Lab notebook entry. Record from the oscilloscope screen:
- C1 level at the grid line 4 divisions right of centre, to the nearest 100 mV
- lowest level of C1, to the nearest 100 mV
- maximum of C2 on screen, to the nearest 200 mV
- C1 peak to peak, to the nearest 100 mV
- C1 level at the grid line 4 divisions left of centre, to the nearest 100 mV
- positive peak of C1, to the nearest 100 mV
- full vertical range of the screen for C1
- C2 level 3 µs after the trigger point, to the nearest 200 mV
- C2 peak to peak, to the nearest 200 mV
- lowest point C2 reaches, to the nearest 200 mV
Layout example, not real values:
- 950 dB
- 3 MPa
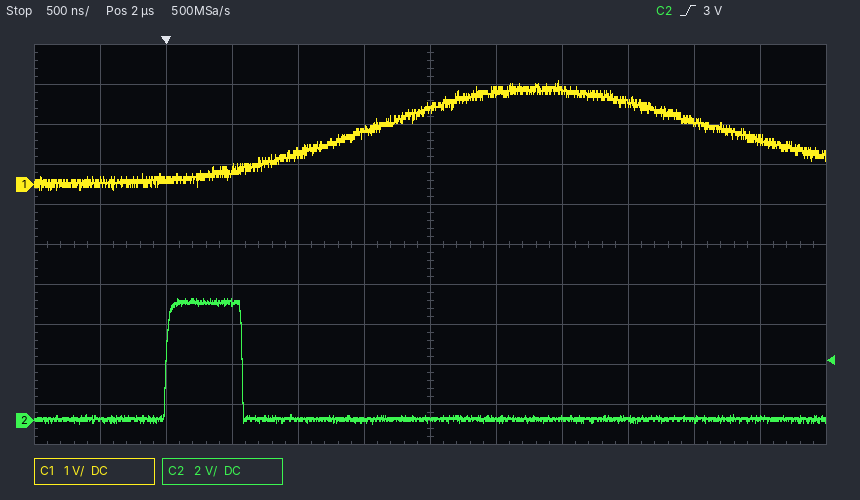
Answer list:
- 1.6 V
- -100 mV
- 6.0 V
- 2.7 V
- 100 mV
- 2.6 V
- 10 V
- 200 mV
- 6.2 V
- -200 mV
